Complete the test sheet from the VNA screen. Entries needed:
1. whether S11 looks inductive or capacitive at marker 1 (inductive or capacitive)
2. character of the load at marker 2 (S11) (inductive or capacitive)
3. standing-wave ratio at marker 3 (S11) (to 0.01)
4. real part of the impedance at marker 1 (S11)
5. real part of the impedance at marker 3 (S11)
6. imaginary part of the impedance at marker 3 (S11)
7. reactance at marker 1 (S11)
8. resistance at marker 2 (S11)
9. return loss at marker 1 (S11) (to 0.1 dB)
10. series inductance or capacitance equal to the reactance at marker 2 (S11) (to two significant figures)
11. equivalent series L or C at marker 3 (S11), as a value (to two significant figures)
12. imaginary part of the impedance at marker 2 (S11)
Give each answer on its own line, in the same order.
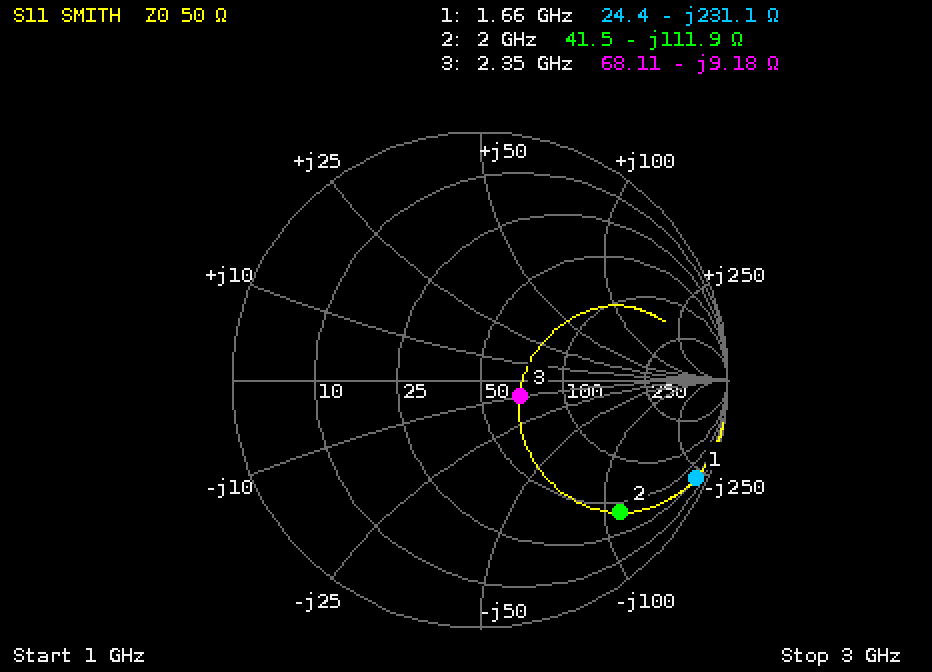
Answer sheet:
capacitive
capacitive
1.41
24.4 Ω
68.11 Ω
-9.18 Ω
-231.1 Ω
41.5 Ω
0.4 dB
710 fF
7.4 pF
-111.9 Ω
